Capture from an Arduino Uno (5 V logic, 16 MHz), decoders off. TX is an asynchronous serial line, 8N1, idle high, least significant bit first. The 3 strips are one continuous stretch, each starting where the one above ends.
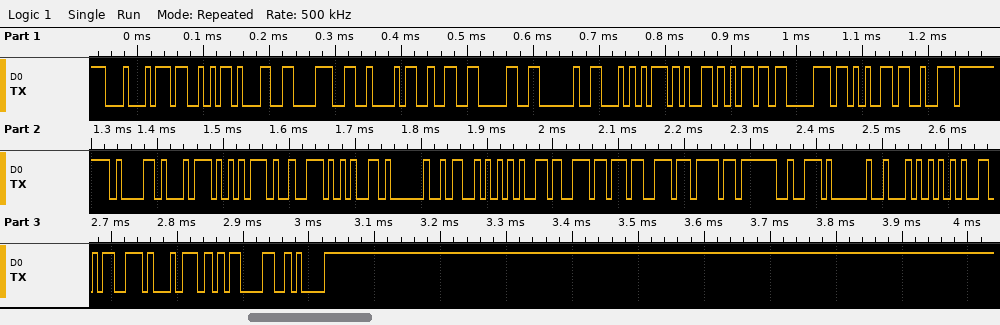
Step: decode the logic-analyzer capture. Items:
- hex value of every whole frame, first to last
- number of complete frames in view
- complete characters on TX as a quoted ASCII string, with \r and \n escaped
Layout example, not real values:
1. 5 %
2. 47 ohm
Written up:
1. 44 53 31 38 42 32 30 20 54 65 6D 70 65 72 61 74 75 72 65 20 53 65 6E 73 6F 72 20 54 65 73 74 0D 0A
2. 33
3. "DS18B20 Temperature Sensor Test\r\n"
